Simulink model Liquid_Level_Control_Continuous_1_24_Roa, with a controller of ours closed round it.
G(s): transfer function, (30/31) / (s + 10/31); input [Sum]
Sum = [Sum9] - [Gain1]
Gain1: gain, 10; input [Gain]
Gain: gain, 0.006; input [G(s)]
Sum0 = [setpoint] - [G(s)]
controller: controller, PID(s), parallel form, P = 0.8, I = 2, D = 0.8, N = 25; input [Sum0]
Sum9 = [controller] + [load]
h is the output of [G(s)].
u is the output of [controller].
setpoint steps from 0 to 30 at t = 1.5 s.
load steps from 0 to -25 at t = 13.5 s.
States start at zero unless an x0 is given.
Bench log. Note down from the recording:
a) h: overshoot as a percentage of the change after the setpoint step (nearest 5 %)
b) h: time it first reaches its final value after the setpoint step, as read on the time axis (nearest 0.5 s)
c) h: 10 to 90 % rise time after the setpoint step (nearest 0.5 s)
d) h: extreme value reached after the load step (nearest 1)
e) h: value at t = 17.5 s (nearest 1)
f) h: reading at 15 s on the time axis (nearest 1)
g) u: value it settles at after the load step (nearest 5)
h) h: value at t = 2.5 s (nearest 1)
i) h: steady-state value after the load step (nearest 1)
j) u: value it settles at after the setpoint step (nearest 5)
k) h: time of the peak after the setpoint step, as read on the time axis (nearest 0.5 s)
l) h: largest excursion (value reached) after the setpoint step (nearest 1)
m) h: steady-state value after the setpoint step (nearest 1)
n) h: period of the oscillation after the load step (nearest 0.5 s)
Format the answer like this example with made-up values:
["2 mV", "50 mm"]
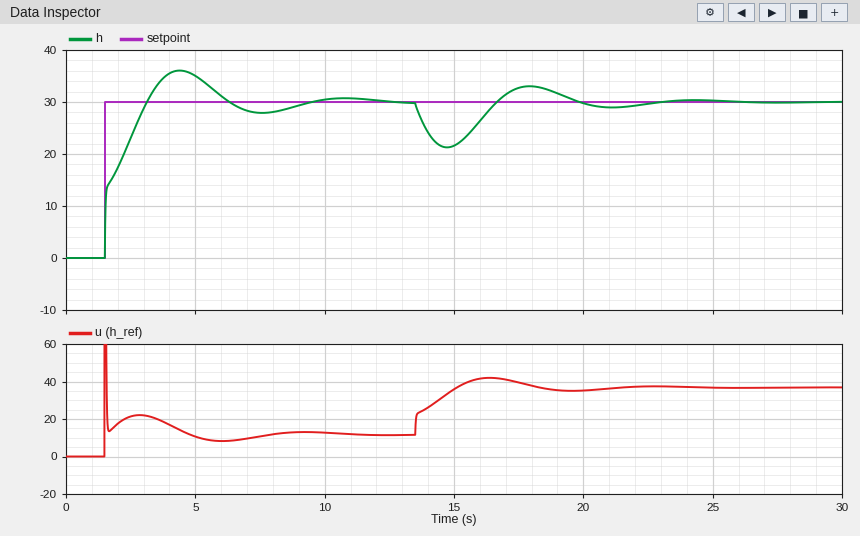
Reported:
["20 %", "3.0 s", "1.5 s", "21", "33", "22", "35", "23", "30", "10", "4.5 s", "36", "30", "6.5 s"]
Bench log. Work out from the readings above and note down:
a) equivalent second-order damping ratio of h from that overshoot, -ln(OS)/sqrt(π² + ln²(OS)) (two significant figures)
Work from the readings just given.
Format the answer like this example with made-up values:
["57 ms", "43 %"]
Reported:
["0.46"]
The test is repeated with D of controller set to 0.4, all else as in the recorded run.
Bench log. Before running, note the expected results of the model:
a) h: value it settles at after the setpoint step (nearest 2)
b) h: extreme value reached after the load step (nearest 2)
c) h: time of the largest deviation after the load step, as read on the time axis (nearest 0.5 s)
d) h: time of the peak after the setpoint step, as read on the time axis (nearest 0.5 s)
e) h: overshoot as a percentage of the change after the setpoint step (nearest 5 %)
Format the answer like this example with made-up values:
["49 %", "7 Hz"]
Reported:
["30", "20", "14.5 s", "4.0 s", "25 %"]
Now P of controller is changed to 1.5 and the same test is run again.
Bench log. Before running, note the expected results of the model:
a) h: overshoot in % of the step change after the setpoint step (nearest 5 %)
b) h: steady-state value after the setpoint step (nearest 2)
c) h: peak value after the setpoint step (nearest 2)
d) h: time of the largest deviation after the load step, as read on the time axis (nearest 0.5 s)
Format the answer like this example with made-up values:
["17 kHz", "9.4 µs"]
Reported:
["10 %", "30", "34", "14.5 s"]
